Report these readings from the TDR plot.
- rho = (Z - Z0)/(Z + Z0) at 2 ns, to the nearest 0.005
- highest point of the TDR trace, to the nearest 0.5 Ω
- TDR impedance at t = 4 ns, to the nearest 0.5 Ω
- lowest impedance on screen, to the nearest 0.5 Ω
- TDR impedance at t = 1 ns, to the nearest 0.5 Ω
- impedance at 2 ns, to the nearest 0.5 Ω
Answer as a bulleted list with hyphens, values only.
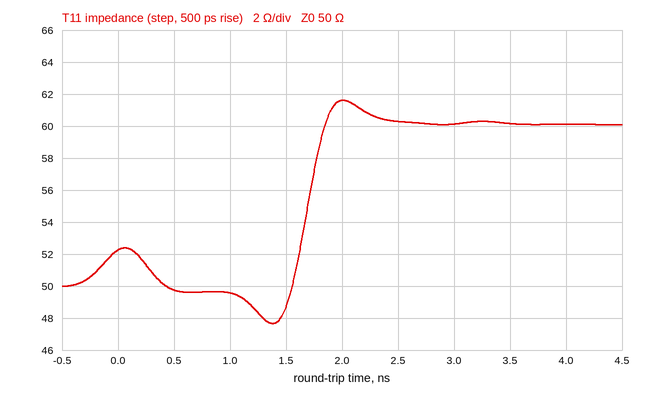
- +0.105
- 61.5 Ω
- 60.0 Ω
- 47.5 Ω
- 49.5 Ω
- 61.5 Ω
